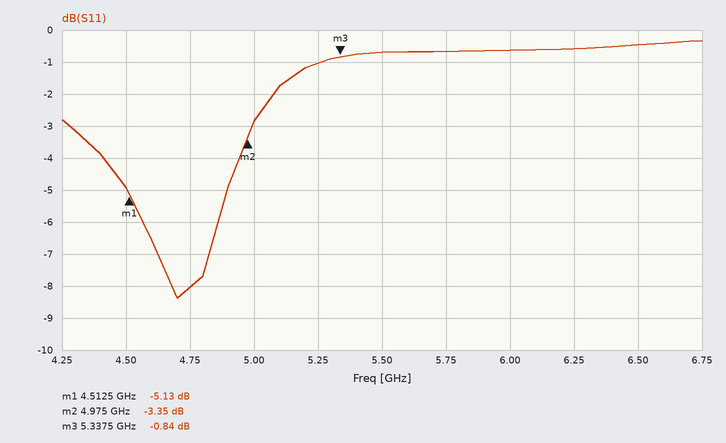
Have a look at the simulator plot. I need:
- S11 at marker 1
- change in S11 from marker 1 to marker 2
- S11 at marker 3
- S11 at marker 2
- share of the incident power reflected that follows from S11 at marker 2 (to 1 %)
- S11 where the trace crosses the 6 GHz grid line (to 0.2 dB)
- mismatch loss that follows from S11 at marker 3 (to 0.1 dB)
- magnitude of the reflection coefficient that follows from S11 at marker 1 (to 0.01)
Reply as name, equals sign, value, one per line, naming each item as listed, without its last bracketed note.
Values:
S11 at marker 1 = -5.13 dB
change in S11 from marker 1 to marker 2 = 1.78 dB
S11 at marker 3 = -0.84 dB
S11 at marker 2 = -3.35 dB
share of the incident power reflected that follows from S11 at marker 2 = 46 %
S11 where the trace crosses the 6 GHz grid line = -0.6 dB
mismatch loss that follows from S11 at marker 3 = 7.5 dB
magnitude of the reflection coefficient that follows from S11 at marker 1 = 0.55
